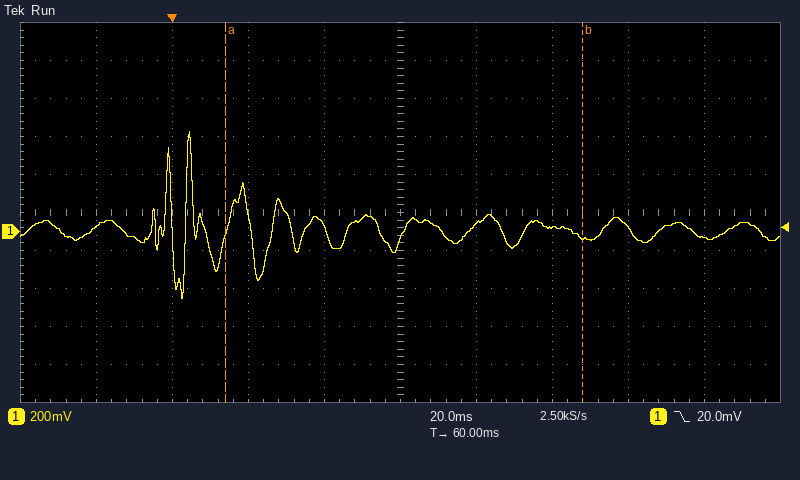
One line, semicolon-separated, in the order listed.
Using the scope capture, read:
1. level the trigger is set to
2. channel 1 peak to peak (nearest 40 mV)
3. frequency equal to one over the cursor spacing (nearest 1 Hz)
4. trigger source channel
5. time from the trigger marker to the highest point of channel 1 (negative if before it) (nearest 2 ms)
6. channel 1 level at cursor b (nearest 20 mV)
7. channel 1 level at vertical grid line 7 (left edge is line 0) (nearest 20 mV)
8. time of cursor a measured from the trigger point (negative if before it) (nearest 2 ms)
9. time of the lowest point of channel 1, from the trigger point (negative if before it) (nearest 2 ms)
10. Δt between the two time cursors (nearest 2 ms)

20.0 mV; 880 mV; 11 Hz; channel 1; +4 ms; -40 mV; 20 mV; +14 ms; +2 ms; 94 ms
